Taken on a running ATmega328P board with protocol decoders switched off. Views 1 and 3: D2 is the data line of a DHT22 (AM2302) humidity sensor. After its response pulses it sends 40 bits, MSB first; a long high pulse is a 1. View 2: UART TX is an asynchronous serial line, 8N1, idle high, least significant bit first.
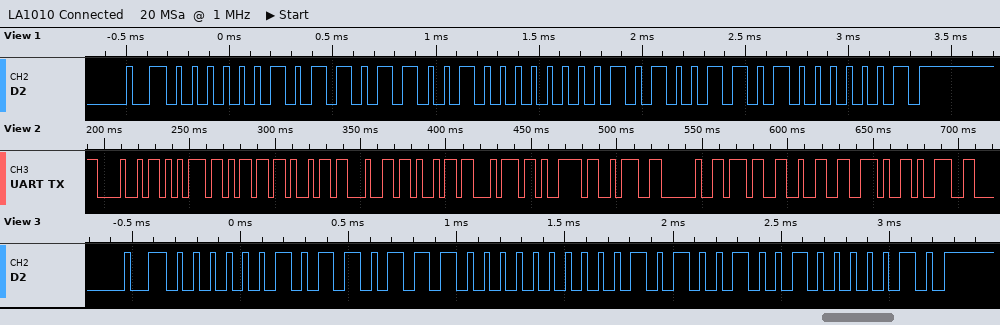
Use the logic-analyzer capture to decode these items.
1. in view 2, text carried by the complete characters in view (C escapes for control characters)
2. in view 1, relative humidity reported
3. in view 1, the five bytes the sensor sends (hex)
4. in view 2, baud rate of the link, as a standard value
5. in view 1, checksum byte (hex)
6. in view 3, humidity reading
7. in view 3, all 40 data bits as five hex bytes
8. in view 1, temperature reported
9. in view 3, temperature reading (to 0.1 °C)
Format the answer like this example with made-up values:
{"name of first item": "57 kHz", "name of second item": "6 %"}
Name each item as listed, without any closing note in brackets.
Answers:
{"in view 2, text carried by the complete characters in view": "\"Humidity: 72.9\"", "in view 1, relative humidity reported": "72.9 %", "in view 1, the five bytes the sensor sends": "02 D9 00 A6 81", "in view 2, baud rate of the link, as a standard value": "300 baud", "in view 1, checksum byte": "0x81", "in view 3, humidity reading": "73.2 %", "in view 3, all 40 data bits as five hex bytes": "02 DC 00 A4 82", "in view 1, temperature reported": "16.6 °C", "in view 3, temperature reading": "16.4 °C"}
